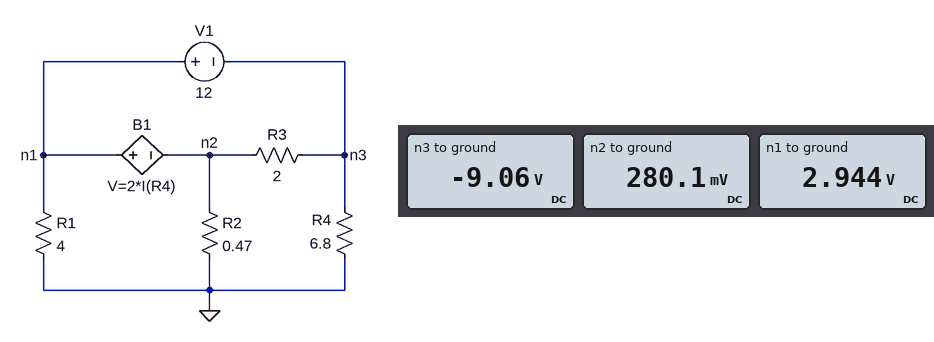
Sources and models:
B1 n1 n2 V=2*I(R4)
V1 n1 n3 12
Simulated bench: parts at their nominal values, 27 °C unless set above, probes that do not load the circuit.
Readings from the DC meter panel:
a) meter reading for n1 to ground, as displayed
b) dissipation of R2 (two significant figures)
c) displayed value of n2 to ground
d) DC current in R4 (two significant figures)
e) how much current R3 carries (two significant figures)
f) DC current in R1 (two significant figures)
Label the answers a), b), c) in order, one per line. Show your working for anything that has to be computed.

a) 2.944 V
b) (280.1 mV)^2 / 470 mΩ = 170 mW
c) 280.1 mV
d) (0 V - (-9.06 V)) / 6.8 Ω = 1.3 A
e) (280.1 mV - (-9.06 V)) / 2 Ω = 4.7 A
f) (2.944 V) / 4 Ω = 740 mA
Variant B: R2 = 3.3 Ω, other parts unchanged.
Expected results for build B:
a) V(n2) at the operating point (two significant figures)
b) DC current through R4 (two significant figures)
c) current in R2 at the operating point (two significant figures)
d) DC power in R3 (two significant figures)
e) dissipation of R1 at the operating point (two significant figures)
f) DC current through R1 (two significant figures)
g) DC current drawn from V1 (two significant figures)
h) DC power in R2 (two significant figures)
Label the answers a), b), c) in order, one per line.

a) 1.1 V
b) 1.2 A
c) 340 mA
d) 45 W
e) 3.2 W
f) 900 mA
g) 6.0 A
h) 380 mW
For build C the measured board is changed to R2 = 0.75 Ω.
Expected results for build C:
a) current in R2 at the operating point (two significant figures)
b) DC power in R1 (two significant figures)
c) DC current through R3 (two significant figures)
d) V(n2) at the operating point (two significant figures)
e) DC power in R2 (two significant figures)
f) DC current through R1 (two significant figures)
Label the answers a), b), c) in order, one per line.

a) 550 mA
b) 2.3 W
c) 4.7 A
d) 420 mV
e) 230 mW
f) 760 mA
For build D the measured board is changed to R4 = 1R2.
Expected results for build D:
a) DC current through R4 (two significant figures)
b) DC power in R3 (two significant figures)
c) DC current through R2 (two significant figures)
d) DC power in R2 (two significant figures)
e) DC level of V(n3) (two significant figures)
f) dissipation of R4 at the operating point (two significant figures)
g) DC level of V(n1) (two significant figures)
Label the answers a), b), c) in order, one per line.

a) 3.5 A
b) 12 W
c) 1.6 A
d) 1.2 W
e) -4.2 V
f) 15 W
g) 7.8 V
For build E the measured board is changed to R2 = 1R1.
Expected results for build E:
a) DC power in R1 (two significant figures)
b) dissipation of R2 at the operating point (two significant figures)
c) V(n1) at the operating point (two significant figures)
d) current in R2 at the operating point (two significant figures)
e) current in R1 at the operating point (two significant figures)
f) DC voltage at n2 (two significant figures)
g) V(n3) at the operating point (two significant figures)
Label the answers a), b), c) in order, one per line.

a) 2.5 W
b) 290 mW
c) 3.2 V
d) 510 mA
e) 790 mA
f) 560 mV
g) -8.8 V
